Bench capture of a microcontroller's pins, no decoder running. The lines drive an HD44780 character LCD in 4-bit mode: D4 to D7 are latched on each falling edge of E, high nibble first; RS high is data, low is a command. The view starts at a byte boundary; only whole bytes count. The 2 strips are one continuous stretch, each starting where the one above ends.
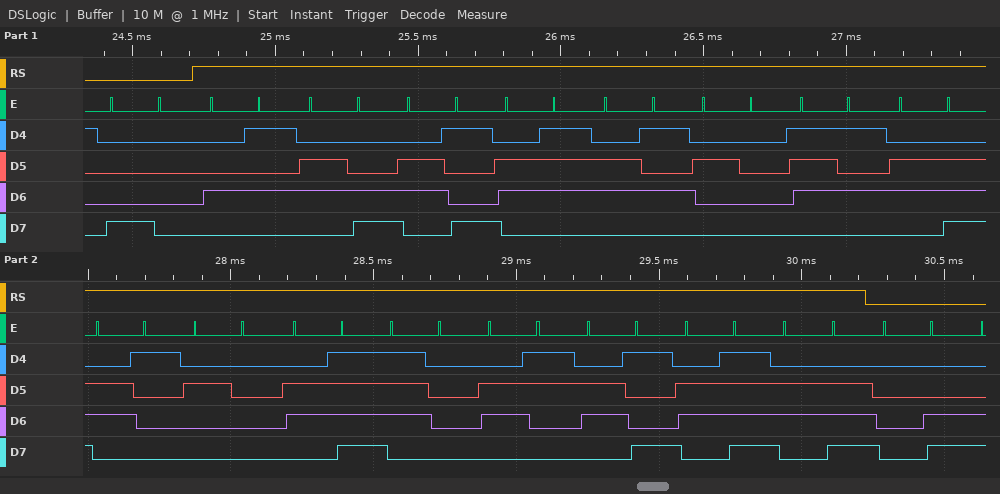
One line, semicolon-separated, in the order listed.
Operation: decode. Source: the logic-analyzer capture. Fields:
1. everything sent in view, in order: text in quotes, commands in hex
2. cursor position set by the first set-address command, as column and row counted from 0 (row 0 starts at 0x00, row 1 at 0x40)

0x80 "Elige una opcion" 0x0C; column 0, row 0
